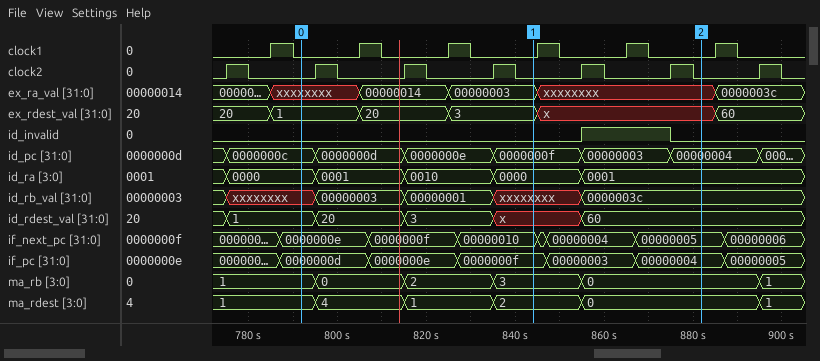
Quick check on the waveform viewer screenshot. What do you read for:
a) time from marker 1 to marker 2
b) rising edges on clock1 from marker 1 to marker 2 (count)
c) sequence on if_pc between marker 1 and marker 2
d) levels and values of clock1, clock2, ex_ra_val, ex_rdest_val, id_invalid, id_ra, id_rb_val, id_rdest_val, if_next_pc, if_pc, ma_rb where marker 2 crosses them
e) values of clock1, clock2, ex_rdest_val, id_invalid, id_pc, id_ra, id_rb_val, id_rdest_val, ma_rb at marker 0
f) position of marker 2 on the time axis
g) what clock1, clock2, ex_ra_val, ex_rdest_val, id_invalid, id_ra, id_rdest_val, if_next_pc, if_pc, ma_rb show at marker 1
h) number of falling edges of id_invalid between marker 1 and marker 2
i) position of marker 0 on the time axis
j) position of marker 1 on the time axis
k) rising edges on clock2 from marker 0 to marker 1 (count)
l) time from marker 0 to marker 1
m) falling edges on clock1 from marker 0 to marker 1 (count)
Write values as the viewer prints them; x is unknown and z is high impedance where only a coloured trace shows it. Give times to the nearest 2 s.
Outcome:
38 s
2
0000000f, 00000003, 00000004
clock1=0, clock2=0, ex_ra_val=xxxxxxxx, ex_rdest_val=x, id_invalid=0, id_ra=0001, id_rb_val=0000003c, id_rdest_val=60, if_next_pc=00000005, if_pc=00000004, ma_rb=0
clock1=0, clock2=0, ex_rdest_val=1, id_invalid=0, id_pc=0000000c, id_ra=0000, id_rb_val=xxxxxxxx, id_rdest_val=1, ma_rb=1
882 s
clock1=0, clock2=0, ex_ra_val=00000003, ex_rdest_val=3, id_invalid=0, id_ra=0000, id_rdest_val=x, if_next_pc=00000010, if_pc=0000000f, ma_rb=3
1
792 s
844 s
3
52 s
2
